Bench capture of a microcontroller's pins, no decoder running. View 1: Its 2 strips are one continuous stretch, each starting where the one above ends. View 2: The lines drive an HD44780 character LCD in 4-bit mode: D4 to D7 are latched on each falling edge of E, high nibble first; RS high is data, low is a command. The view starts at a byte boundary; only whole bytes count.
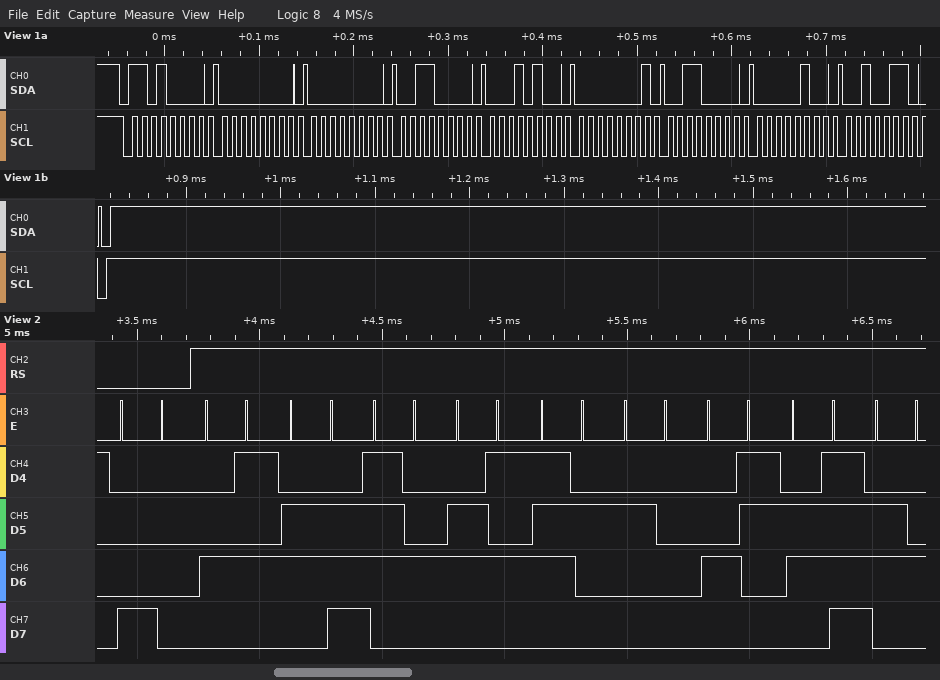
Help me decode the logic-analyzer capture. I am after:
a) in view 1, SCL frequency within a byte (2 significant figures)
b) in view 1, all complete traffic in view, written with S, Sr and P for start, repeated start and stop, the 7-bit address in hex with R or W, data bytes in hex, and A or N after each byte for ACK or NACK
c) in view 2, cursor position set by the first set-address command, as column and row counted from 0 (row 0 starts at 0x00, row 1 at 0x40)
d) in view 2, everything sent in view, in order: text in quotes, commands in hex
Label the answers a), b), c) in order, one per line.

a) 100 kHz
b) S 68W A 00 A 00 A 30 A 14 A 01 A 30 A 04 A 26 A P
c) column 0, row 0
d) 0x80 "Enter Cod"
